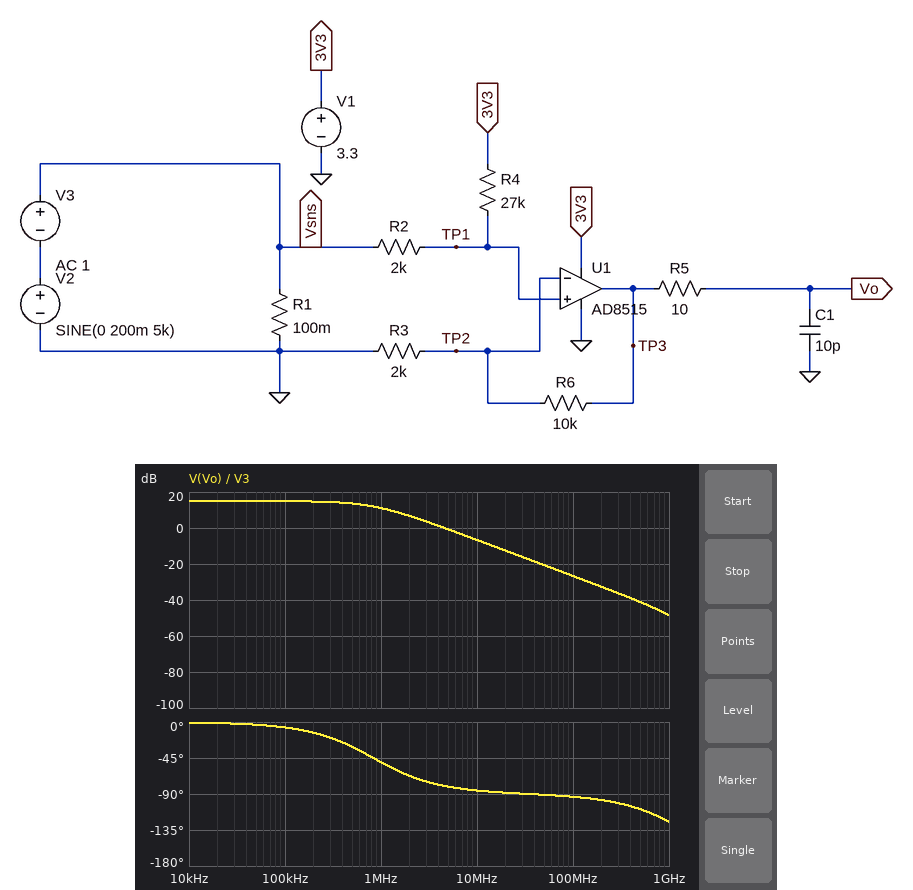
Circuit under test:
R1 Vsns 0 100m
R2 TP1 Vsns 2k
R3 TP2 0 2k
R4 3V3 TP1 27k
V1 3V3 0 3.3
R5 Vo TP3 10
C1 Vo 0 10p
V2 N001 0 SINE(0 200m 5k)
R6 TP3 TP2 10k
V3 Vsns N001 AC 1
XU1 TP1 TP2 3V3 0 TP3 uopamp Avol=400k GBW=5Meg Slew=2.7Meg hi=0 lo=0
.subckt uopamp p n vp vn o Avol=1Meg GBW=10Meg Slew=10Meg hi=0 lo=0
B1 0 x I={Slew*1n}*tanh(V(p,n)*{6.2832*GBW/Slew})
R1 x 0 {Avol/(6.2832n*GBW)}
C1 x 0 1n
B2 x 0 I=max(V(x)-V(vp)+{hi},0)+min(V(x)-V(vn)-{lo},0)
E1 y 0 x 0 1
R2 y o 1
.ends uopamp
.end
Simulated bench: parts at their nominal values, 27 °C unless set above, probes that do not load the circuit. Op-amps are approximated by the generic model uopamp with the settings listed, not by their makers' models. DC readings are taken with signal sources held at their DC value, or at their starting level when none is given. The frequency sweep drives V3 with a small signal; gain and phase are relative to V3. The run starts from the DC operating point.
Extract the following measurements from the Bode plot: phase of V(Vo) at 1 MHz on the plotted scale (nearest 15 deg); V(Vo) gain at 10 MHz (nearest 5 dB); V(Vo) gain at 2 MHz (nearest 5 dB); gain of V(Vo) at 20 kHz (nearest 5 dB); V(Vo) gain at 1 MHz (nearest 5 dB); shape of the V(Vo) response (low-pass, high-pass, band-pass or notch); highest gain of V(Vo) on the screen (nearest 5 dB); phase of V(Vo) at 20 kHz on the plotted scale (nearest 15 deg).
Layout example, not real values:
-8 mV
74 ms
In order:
-45 deg
-5 dB
5 dB
15 dB
10 dB
low-pass
15 dB
0 deg
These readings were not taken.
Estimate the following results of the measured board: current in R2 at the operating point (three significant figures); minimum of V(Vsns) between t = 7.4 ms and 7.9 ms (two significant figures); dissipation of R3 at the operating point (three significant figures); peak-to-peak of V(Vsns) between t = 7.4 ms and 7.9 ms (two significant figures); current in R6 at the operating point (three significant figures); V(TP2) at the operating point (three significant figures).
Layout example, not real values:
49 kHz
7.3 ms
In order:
114 µA
-200 mV
25.9 µW
400 mV
114 µA
228 mV
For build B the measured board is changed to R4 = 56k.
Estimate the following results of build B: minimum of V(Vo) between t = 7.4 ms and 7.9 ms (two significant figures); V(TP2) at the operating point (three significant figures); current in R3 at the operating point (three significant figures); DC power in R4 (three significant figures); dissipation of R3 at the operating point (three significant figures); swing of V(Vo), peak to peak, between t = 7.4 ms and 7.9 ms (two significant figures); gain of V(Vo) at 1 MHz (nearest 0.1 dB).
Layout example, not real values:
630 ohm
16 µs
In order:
-2.0 mV
114 mV
56.9 µA
181 µW
6.47 µW
1.8 V
11.4 dB
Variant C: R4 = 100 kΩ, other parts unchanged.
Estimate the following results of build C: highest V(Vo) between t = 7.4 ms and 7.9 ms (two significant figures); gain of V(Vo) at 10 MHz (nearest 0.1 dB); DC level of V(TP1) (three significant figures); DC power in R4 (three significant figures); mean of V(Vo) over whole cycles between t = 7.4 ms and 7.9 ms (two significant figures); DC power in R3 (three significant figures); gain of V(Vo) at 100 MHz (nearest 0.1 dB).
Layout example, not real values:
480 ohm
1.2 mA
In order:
1.6 V
-6.2 dB
64.7 mV
105 µW
590 mV
2.09 µW
-26.2 dB
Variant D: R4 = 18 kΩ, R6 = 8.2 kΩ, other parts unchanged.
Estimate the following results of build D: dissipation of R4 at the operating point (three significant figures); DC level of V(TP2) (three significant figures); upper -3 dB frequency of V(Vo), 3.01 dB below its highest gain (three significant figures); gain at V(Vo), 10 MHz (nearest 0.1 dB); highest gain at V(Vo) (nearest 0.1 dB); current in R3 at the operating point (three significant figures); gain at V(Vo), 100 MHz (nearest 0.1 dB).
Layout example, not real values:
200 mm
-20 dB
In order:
490 µW
330 mV
980 kHz
-7.0 dB
13.2 dB
165 µA
-27.0 dB
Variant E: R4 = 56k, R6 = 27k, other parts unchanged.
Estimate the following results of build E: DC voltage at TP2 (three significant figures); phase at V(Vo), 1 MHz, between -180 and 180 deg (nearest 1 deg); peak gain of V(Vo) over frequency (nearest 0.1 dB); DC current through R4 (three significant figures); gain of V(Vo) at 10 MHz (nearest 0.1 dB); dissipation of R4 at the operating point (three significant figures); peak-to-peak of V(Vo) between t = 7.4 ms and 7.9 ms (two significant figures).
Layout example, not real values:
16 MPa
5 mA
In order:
114 mV
-71 deg
22.9 dB
56.9 µA
-6.3 dB
181 µW
3.3 V
